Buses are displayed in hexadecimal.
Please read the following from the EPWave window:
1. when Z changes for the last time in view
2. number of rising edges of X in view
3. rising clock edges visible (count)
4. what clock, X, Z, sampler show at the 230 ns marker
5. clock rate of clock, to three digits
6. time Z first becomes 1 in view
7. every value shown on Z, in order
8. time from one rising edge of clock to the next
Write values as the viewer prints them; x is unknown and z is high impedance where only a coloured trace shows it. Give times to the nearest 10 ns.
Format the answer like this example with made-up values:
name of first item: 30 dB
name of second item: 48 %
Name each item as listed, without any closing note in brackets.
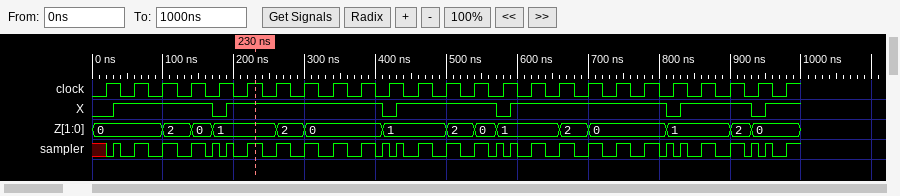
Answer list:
when Z changes for the last time in view: 930 ns
number of rising edges of X in view: 6
rising clock edges visible: 25
what clock, X, Z, sampler show at the 230 ns marker: clock=1, X=1, Z=1, sampler=1
clock rate of clock, to three digits: 25.0 MHz
time Z first becomes 1 in view: 170 ns
every value shown on Z, in order: 0, 2, 0, 1, 2, 0, 1, 2, 0, 1, 2, 0, 1, 2, 0
time from one rising edge of clock to the next: 40 ns
